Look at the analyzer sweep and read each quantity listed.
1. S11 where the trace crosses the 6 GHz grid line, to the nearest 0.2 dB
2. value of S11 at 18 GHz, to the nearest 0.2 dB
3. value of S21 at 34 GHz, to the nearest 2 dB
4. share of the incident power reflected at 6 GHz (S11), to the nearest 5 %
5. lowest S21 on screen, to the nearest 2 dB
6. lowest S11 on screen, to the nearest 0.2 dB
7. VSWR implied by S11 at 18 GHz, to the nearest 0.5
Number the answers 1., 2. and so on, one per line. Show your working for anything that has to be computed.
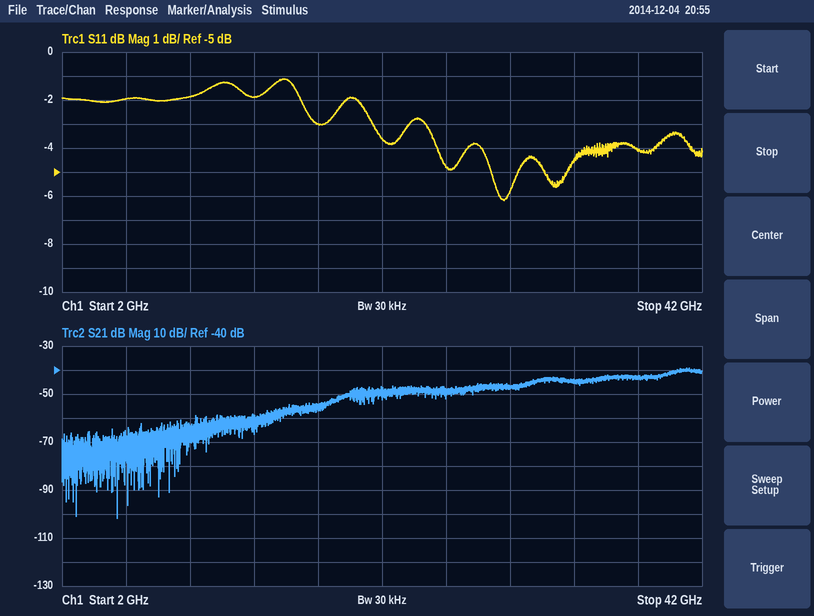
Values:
1. -2.0 dB
2. -3.0 dB
3. -44 dB
4. 10^(-2/10) ≈ 63.1 %, so 65 % to the nearest 5 %
5. -102 dB
6. -6.2 dB
7. |Γ| = 10^(-3/20) = 0.7079; VSWR = (1 + 0.7079)/(1 − 0.7079) ≈ 5.85, so 6.0 to the nearest 0.5
